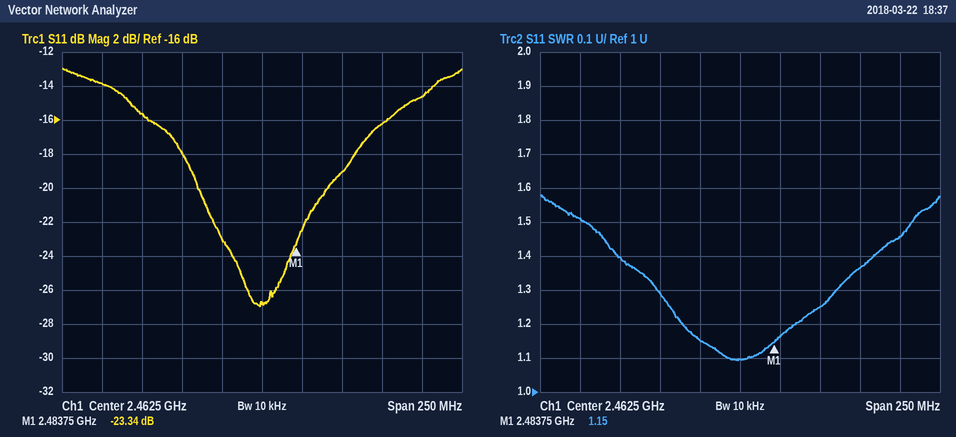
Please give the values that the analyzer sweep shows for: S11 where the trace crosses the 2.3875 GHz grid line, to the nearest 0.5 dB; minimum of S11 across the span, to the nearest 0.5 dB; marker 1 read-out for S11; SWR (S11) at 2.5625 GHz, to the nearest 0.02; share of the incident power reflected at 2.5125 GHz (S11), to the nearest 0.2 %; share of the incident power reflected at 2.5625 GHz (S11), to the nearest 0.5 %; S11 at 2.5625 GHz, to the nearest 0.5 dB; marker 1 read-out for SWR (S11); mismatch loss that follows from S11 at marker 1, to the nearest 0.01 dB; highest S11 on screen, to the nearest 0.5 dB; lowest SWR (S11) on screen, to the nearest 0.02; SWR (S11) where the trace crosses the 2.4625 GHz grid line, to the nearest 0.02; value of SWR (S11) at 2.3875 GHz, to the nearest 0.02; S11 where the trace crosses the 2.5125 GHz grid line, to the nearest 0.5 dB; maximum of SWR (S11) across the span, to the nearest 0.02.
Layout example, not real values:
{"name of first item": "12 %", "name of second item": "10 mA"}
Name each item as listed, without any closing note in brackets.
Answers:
{"S11 where the trace crosses the 2.3875 GHz grid line, to the nearest 0.5 dB": "-15.5 dB", "minimum of S11 across the span, to the nearest 0.5 dB": "-27.0 dB", "marker 1 read-out for S11": "-23.34 dB", "SWR (S11) at 2.5625 GHz, to the nearest 0.02": "1.46", "share of the incident power reflected at 2.5125 GHz (S11), to the nearest 0.2 %": "1.2 %", "share of the incident power reflected at 2.5625 GHz (S11), to the nearest 0.5 %": "3.5 %", "S11 at 2.5625 GHz, to the nearest 0.5 dB": "-14.5 dB", "marker 1 read-out for SWR": "1.15", "mismatch loss that follows from S11 at marker 1, to the nearest 0.01 dB": "0.02 dB", "highest S11 on screen, to the nearest 0.5 dB": "-13.0 dB", "lowest SWR (S11) on screen, to the nearest 0.02": "1.10", "SWR (S11) where the trace crosses the 2.4625 GHz grid line, to the nearest 0.02": "1.10", "value of SWR (S11) at 2.3875 GHz, to the nearest 0.02": "1.40", "S11 where the trace crosses the 2.5125 GHz grid line, to the nearest 0.5 dB": "-19.0 dB", "maximum of SWR (S11) across the span, to the nearest 0.02": "1.58"}
